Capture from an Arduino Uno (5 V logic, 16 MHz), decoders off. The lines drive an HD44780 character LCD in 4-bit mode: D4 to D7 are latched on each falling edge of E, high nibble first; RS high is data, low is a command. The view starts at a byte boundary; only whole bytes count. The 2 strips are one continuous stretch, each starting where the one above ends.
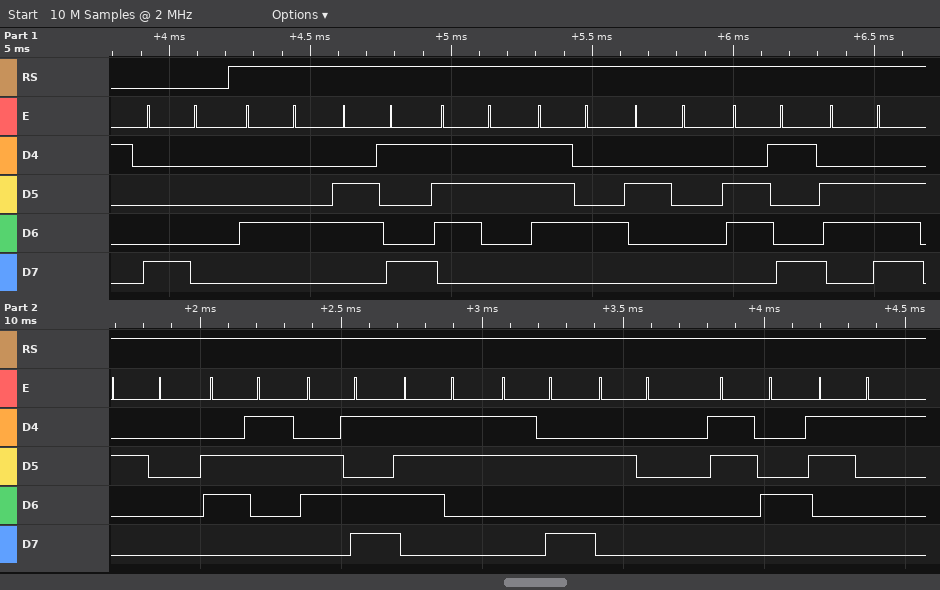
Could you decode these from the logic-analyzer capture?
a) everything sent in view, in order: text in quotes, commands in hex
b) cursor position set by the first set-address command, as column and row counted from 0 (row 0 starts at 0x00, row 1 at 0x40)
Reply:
0x80 "Dist in cms: 41"
column 0, row 0
